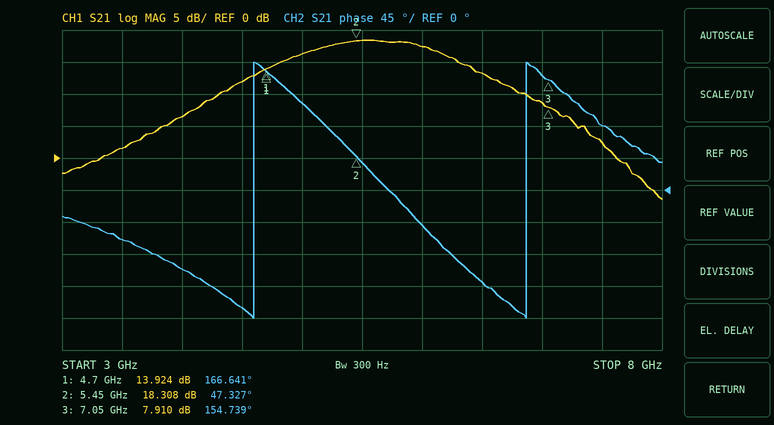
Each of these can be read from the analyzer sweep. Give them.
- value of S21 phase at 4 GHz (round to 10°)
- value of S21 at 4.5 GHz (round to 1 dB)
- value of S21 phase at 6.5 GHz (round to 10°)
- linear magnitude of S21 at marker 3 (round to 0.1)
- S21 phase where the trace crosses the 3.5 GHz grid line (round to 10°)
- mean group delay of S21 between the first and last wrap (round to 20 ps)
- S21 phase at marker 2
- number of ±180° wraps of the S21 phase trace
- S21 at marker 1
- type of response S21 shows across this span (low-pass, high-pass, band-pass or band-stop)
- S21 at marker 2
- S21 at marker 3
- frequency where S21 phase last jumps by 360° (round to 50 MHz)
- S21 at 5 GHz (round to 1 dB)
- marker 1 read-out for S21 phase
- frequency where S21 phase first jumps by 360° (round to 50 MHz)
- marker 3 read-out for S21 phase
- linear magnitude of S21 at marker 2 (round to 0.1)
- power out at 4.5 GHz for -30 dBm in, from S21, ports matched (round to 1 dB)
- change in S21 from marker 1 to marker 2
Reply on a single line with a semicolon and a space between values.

-110°; 12 dB; -130°; 2.5; -70°; 440 ps; 47.327°; 2; 13.924 dB; band-pass; 18.308 dB; 7.910 dB; 6.85 GHz; 16 dB; 166.641°; 4.60 GHz; 154.739°; 8.2; -18 dBm; 4.384 dB
